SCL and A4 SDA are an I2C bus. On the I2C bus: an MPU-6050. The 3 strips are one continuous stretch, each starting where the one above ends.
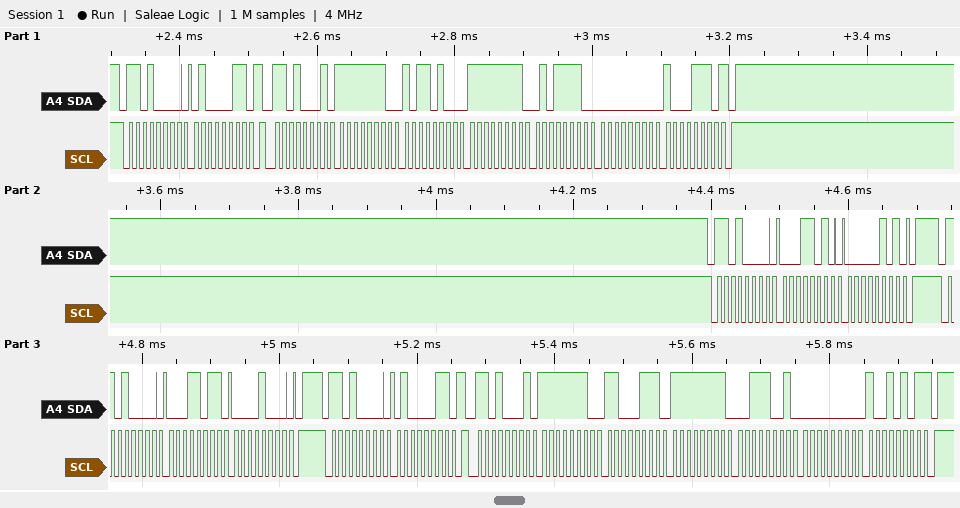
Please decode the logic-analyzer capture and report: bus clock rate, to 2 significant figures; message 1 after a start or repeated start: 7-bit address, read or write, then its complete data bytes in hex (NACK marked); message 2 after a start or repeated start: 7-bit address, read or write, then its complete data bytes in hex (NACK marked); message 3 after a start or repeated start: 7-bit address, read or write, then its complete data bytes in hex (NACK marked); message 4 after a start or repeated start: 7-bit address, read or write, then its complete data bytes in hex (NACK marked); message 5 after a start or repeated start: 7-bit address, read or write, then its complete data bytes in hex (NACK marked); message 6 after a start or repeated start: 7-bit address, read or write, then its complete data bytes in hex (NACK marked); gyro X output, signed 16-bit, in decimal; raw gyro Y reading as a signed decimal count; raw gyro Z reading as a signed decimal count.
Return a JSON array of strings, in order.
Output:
["100 kHz", "0x68 write: 43", "0x68 read: FE B4 FF 5E 00 8E NACK", "0x68 write: 1A 05", "0x68 write: 1B 08", "0x68 write: 43", "0x68 read: FE C7 FF 39 00 95 NACK", "-332", "-162", "142"]
